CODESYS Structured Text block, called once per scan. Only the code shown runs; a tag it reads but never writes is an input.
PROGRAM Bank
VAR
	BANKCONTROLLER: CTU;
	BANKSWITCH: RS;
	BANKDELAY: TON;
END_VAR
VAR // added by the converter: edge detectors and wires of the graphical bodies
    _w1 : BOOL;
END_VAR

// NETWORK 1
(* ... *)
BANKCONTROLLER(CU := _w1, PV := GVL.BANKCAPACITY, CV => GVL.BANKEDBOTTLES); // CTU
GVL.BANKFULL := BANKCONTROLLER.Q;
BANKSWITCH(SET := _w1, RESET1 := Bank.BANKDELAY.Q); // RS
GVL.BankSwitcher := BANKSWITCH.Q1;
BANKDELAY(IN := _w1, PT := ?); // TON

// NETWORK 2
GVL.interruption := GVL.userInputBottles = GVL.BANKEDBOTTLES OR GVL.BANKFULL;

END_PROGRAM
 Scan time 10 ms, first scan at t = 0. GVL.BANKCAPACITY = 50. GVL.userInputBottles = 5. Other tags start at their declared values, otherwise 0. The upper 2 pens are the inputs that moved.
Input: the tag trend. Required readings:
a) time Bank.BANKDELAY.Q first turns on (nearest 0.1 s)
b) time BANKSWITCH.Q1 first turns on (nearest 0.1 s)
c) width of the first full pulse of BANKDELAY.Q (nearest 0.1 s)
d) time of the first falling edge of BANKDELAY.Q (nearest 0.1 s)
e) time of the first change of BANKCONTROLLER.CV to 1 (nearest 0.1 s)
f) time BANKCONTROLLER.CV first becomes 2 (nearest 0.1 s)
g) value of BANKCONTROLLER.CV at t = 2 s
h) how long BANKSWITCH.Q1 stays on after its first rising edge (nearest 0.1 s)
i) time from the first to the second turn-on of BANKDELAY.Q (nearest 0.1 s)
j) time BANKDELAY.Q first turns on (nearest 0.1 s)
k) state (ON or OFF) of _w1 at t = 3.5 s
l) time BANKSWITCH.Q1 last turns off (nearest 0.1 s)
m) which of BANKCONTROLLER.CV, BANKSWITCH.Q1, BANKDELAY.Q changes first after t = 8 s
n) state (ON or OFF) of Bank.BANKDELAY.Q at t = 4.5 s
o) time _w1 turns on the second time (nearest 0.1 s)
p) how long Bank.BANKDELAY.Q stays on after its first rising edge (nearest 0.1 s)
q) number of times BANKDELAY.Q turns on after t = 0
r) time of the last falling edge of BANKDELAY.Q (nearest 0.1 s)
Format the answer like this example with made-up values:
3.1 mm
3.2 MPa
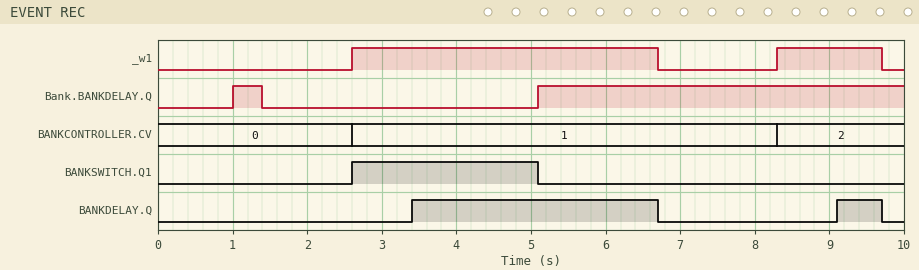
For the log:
1.0 s
2.6 s
3.3 s
6.7 s
2.6 s
8.3 s
0
2.5 s
5.7 s
3.4 s
ON
5.1 s
BANKCONTROLLER.CV
OFF
8.3 s
0.4 s
2
9.7 s
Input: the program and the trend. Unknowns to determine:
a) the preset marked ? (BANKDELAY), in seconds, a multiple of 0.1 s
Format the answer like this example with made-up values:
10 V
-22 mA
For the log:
0.8 s
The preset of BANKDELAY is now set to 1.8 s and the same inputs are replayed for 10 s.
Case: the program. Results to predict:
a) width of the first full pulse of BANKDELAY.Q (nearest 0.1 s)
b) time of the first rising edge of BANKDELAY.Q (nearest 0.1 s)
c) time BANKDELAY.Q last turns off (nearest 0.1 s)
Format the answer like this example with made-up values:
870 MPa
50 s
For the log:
2.3 s
4.4 s
6.7 s
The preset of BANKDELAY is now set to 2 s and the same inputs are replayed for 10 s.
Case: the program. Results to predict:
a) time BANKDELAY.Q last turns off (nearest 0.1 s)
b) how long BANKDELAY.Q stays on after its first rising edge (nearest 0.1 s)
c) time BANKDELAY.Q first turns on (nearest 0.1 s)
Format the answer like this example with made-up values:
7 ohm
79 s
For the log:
6.7 s
2.1 s
4.6 s
